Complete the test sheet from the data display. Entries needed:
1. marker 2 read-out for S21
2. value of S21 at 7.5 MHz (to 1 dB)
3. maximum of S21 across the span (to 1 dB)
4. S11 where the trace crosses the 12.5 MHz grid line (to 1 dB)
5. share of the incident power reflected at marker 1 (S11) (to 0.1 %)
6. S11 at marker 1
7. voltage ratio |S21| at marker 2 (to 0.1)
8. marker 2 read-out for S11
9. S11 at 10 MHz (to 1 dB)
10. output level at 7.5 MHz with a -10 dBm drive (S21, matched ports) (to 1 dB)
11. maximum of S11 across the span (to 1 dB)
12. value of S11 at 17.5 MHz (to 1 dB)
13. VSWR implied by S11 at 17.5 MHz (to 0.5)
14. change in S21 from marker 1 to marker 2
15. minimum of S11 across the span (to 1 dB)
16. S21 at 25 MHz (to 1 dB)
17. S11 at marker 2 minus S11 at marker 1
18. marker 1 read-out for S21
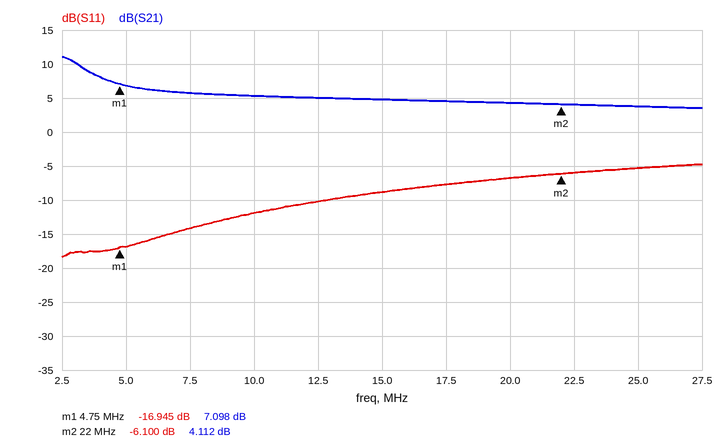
4.112 dB
6 dB
11 dB
-10 dB
2.0 %
-16.945 dB
1.6
-6.100 dB
-12 dB
-4 dBm
-5 dB
-8 dB
2.5
-2.986 dB
-18 dB
4 dB
10.845 dB
7.098 dB
